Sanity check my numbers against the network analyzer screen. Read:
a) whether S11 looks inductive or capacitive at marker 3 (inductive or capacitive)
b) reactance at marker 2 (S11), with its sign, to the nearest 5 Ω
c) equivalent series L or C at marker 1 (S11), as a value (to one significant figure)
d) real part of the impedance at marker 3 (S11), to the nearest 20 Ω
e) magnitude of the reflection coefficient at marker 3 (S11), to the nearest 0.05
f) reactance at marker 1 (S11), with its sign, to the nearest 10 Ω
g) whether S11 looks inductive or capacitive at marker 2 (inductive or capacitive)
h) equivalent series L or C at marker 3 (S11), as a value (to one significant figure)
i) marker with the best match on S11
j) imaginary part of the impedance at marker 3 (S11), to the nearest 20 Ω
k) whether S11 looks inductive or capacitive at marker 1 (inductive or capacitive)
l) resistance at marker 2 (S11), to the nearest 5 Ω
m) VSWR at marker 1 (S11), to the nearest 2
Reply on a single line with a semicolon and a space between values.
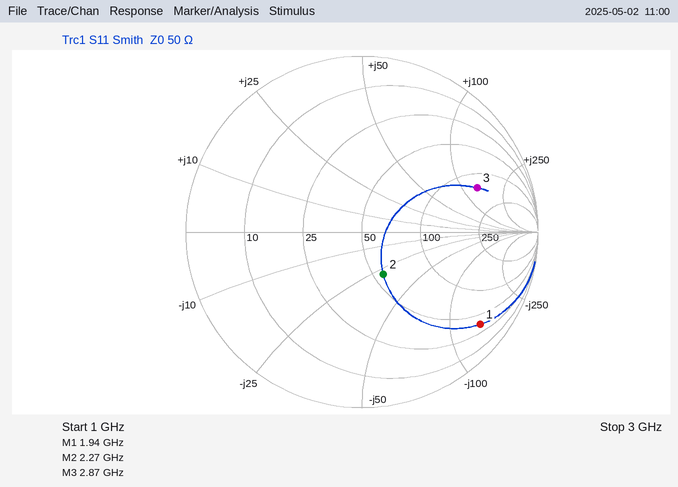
inductive; -30 Ω; 600 fF; 140 Ω; 0.70; -140 Ω; capacitive; 8 nH; marker 2; +140 Ω; capacitive; 55 Ω; 12
